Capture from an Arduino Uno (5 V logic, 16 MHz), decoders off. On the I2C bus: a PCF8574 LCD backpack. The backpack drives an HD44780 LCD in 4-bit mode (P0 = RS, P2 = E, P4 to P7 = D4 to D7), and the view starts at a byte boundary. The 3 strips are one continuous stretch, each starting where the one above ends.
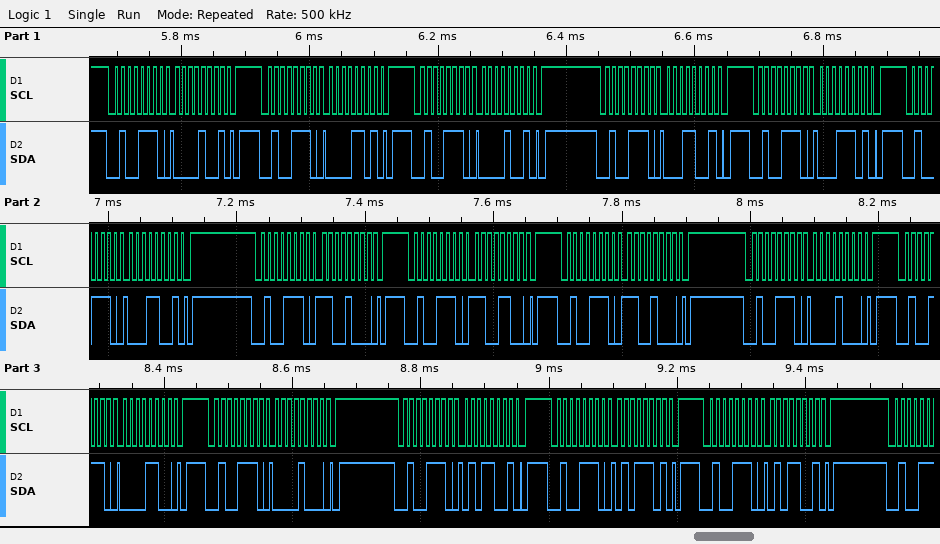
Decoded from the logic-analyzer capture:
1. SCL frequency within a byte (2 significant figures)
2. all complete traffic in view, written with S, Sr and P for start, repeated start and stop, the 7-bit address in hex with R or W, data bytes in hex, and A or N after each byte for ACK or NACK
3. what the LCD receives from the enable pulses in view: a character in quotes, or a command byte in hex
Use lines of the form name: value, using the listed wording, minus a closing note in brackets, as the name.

SCL frequency within a byte: 100 kHz
all complete traffic in view, written with S, Sr and P for start, repeated start and stop, the 7-bit address in hex with R or W, data bytes in hex, and A or N after each byte for ACK or NACK: S 27W A 09 A P S 27W A 0D A P S 27W A 09 A P S 27W A 19 A P S 27W A 1D A P S 27W A 19 A P S 27W A C8 A P S 27W A CC A P S 27W A C8 A P S 27W A 08 A P S 27W A 0C A P S 27W A 08 A P S 27W A 59 A P S 27W A 5D A P S 27W A 59 A P
what the LCD receives from the enable pulses in view: a character in quotes, or a command byte in hex: data 0x01 0xC0
